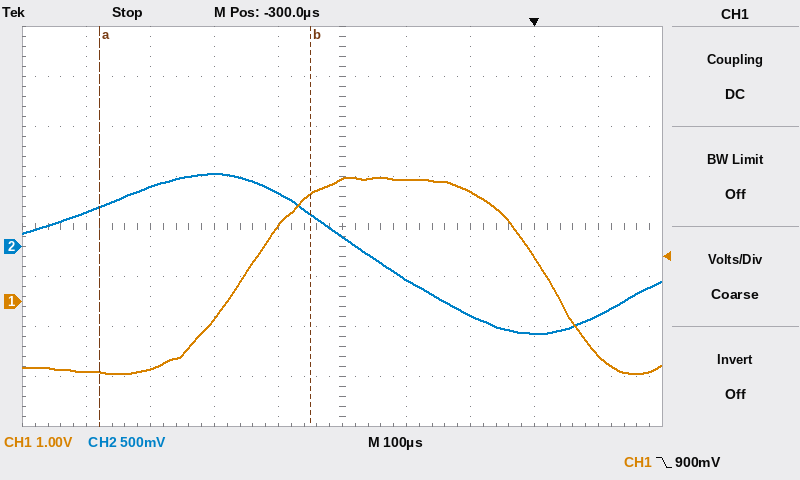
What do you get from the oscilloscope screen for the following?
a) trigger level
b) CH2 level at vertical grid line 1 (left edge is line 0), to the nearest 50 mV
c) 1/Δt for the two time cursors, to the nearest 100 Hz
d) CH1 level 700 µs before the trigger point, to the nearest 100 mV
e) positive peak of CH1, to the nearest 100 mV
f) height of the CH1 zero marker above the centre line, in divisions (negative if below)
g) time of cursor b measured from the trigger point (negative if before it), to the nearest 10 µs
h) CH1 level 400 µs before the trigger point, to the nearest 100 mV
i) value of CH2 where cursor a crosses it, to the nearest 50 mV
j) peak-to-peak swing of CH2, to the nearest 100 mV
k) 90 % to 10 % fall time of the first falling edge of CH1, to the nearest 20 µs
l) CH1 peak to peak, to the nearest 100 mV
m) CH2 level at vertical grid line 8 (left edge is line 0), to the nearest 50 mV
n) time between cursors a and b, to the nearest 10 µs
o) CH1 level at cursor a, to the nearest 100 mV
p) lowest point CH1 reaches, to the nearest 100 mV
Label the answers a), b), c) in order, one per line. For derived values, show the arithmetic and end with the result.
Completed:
a) 900 mV
b) 350 mV
c) 1 / 330 µs ≈ 3.0 kHz
d) -1.4 V
e) 2.5 V
f) -1.5 div
g) -350 µs
h) 1.5 V
i) 400 mV
j) 1.60 V
k) 180 µs
l) 2.5 V − (-1.4 V) = 3.9 V
m) -850 mV
n) 330 µs
o) -1.4 V
p) -1.4 V
